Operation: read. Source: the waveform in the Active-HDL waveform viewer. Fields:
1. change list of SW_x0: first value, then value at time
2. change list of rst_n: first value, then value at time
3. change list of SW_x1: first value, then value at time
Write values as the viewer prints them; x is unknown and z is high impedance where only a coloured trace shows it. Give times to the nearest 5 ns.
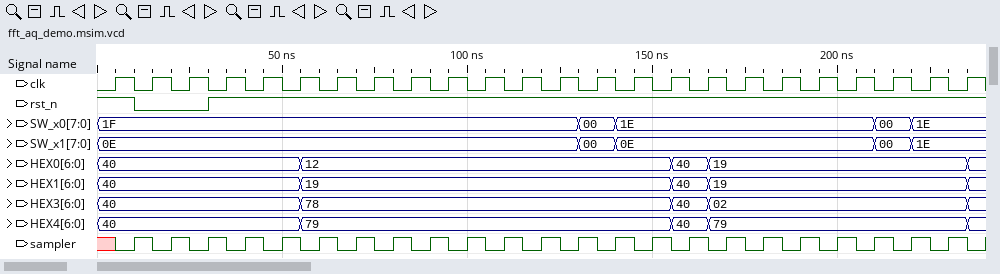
1F, 00 at 130 ns, 1E at 140 ns, 00 at 210 ns, 1E at 220 ns
1, 0 at 10 ns, 1 at 30 ns
0E, 00 at 130 ns, 0E at 140 ns, 00 at 210 ns, 1E at 220 ns
